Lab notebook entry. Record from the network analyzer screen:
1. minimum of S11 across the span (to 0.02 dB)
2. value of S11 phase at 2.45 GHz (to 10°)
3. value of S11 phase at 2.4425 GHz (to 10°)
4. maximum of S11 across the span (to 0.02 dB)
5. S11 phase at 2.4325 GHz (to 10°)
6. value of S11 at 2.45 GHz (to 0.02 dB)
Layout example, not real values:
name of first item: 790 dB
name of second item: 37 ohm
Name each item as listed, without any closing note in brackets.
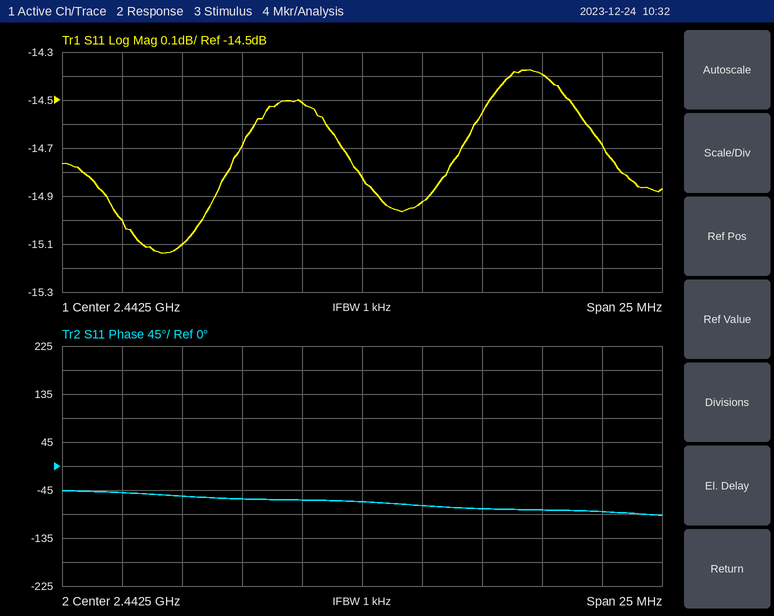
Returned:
minimum of S11 across the span: -15.14 dB
value of S11 phase at 2.45 GHz: -80°
value of S11 phase at 2.4425 GHz: -70°
maximum of S11 across the span: -14.38 dB
S11 phase at 2.4325 GHz: -50°
value of S11 at 2.45 GHz: -14.40 dB
